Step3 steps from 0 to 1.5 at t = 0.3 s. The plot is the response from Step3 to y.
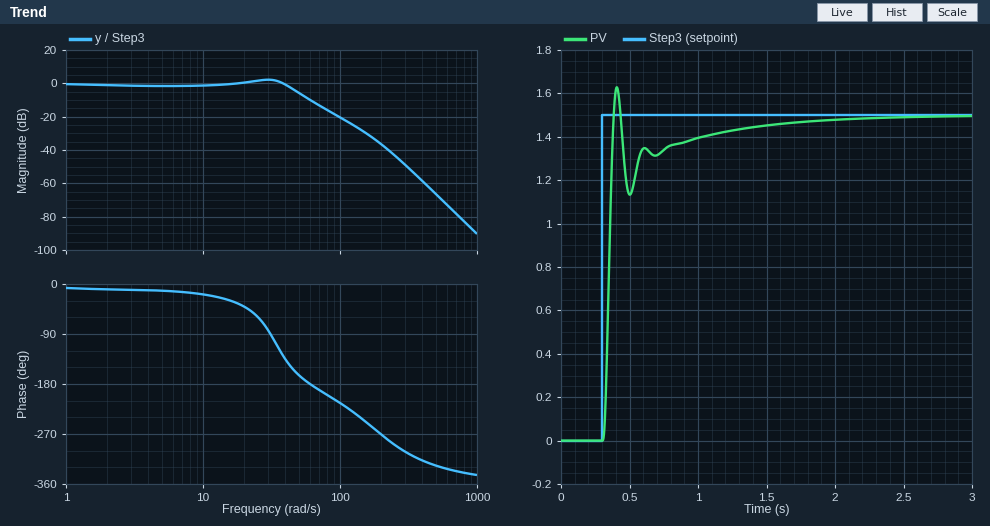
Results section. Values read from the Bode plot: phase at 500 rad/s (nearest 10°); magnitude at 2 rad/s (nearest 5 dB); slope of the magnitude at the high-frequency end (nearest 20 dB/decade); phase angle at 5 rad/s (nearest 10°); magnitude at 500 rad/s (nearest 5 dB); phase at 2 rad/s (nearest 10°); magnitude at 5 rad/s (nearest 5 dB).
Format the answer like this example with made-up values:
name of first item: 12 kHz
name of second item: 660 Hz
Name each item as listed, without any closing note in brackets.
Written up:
phase at 500 rad/s: -330°
magnitude at 2 rad/s: 0 dB
slope of the magnitude at the high-frequency end: -80 dB/decade
phase angle at 5 rad/s: -10°
magnitude at 500 rad/s: -65 dB
phase at 2 rad/s: -10°
magnitude at 5 rad/s: 0 dB
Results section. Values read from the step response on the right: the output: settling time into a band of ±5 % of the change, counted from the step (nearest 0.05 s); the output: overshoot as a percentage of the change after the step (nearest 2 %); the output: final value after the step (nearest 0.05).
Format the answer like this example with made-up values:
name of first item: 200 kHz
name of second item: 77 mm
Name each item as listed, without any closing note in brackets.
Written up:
the output: settling time into a band of ±5 % of the change, counted from the step: 0.90 s
the output: overshoot as a percentage of the change after the step: 8 %
the output: final value after the step: 1.50
